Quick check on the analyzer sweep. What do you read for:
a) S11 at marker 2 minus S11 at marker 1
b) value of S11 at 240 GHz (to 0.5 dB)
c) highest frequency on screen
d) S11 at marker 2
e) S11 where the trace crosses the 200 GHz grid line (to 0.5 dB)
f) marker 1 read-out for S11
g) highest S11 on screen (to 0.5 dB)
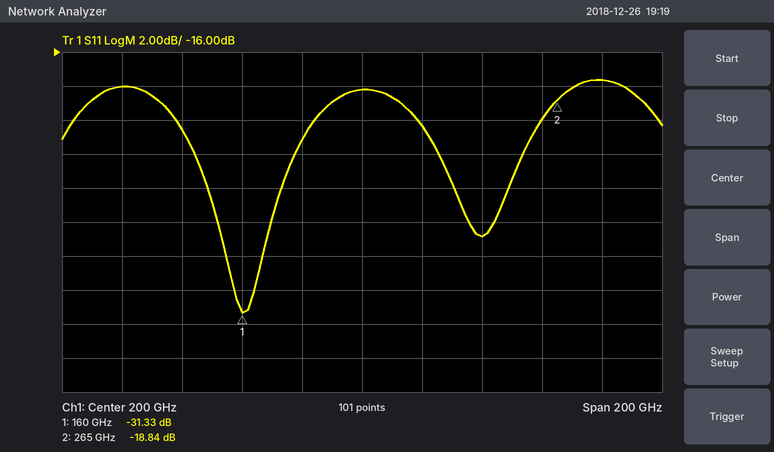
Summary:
12.49 dB
-27.0 dB
300 GHz
-18.84 dB
-18.0 dB
-31.33 dB
-17.5 dB
